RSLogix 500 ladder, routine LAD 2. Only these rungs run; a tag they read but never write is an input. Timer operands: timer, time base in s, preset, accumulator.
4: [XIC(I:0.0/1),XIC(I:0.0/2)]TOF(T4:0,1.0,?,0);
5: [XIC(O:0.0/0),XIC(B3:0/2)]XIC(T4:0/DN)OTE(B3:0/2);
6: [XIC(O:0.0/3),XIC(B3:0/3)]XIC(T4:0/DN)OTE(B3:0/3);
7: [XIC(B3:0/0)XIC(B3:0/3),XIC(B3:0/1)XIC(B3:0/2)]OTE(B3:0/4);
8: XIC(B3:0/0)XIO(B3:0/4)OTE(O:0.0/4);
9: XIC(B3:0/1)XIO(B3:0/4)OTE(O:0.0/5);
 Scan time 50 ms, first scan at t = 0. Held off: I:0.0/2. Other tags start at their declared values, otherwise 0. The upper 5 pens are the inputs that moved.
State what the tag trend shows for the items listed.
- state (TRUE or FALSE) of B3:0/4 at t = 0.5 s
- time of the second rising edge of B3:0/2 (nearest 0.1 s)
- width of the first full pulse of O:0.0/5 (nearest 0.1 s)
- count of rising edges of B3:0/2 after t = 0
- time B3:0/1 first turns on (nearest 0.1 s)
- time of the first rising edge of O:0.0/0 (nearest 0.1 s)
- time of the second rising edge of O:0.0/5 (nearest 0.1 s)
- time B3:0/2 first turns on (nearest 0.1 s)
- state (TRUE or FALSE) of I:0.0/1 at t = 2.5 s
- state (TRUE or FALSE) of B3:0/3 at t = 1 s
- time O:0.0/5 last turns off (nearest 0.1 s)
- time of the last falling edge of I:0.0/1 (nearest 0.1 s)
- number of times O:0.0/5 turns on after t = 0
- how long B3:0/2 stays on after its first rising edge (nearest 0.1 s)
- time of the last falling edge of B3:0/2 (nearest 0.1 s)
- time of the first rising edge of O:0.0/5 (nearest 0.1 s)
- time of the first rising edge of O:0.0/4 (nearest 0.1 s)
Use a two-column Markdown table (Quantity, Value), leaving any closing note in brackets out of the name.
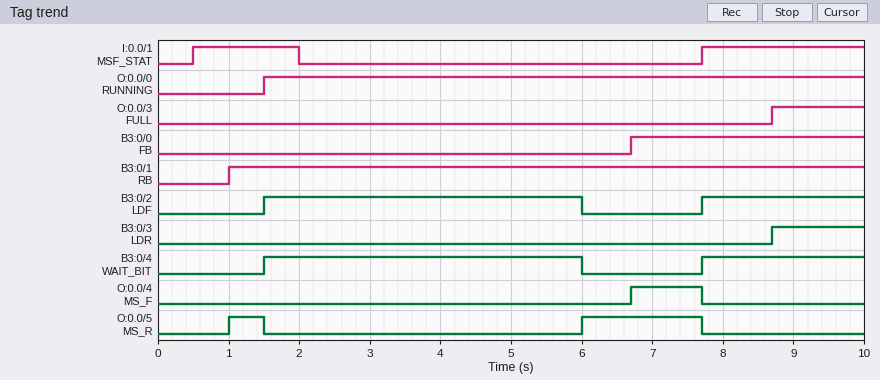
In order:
| Quantity | Value |
|---|---|
| state (TRUE or FALSE) of B3:0/4 at t = 0.5 s | FALSE |
| time of the second rising edge of B3:0/2 | 7.7 s |
| width of the first full pulse of O:0.0/5 | 0.5 s |
| count of rising edges of B3:0/2 after t = 0 | 2 |
| time B3:0/1 first turns on | 1.0 s |
| time of the first rising edge of O:0.0/0 | 1.5 s |
| time of the second rising edge of O:0.0/5 | 6.0 s |
| time B3:0/2 first turns on | 1.5 s |
| state (TRUE or FALSE) of I:0.0/1 at t = 2.5 s | FALSE |
| state (TRUE or FALSE) of B3:0/3 at t = 1 s | FALSE |
| time O:0.0/5 last turns off | 7.7 s |
| time of the last falling edge of I:0.0/1 | 2.0 s |
| number of times O:0.0/5 turns on after t = 0 | 2 |
| how long B3:0/2 stays on after its first rising edge | 4.5 s |
| time of the last falling edge of B3:0/2 | 6.0 s |
| time of the first rising edge of O:0.0/5 | 1.0 s |
| time of the first rising edge of O:0.0/4 | 6.7 s |
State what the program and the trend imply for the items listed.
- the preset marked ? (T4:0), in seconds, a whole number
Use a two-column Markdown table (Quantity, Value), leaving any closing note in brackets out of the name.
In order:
| Quantity | Value |
|---|---|
| the preset marked ? (T4:0), in seconds, a whole number | 4 s |
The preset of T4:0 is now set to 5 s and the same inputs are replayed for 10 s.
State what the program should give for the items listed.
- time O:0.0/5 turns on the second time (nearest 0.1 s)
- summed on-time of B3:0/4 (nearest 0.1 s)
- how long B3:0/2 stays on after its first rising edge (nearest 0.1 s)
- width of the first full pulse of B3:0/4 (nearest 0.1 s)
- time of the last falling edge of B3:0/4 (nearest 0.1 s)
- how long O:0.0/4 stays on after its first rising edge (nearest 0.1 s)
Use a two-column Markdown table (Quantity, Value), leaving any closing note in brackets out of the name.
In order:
| Quantity | Value |
|---|---|
| time O:0.0/5 turns on the second time | 7.0 s |
| summed on-time of B3:0/4 | 7.8 s |
| how long B3:0/2 stays on after its first rising edge | 5.5 s |
| width of the first full pulse of B3:0/4 | 5.5 s |
| time of the last falling edge of B3:0/4 | 7.0 s |
| how long O:0.0/4 stays on after its first rising edge | 0.7 s |
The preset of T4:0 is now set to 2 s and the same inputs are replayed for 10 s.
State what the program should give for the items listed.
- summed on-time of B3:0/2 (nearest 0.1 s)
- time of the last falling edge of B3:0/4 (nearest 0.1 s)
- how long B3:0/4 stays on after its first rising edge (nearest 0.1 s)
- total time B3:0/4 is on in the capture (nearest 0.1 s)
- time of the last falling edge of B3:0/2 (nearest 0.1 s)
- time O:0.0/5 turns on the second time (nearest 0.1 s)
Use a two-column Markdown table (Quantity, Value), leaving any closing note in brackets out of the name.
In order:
| Quantity | Value |
|---|---|
| summed on-time of B3:0/2 | 4.8 s |
| time of the last falling edge of B3:0/4 | 4.0 s |
| how long B3:0/4 stays on after its first rising edge | 2.5 s |
| total time B3:0/4 is on in the capture | 4.8 s |
| time of the last falling edge of B3:0/2 | 4.0 s |
| time O:0.0/5 turns on the second time | 4.0 s |
